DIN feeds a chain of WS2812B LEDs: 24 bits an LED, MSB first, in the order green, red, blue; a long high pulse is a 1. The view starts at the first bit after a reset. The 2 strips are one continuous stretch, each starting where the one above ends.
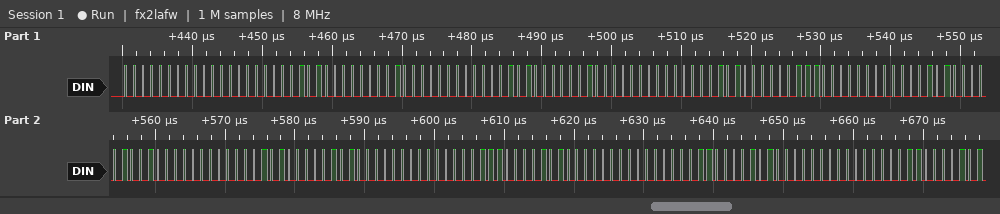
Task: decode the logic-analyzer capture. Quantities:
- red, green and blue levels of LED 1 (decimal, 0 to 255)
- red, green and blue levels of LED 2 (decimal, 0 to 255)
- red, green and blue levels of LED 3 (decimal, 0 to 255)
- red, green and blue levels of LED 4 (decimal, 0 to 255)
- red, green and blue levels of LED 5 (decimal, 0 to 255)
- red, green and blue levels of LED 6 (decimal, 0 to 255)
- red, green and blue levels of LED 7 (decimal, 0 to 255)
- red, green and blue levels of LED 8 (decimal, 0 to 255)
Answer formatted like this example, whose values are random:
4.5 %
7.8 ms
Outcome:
0, 0, 10
0, 1, 10
0, 4, 10
0, 7, 10
0, 9, 10
0, 10, 7
0, 10, 3
0, 10, 3
